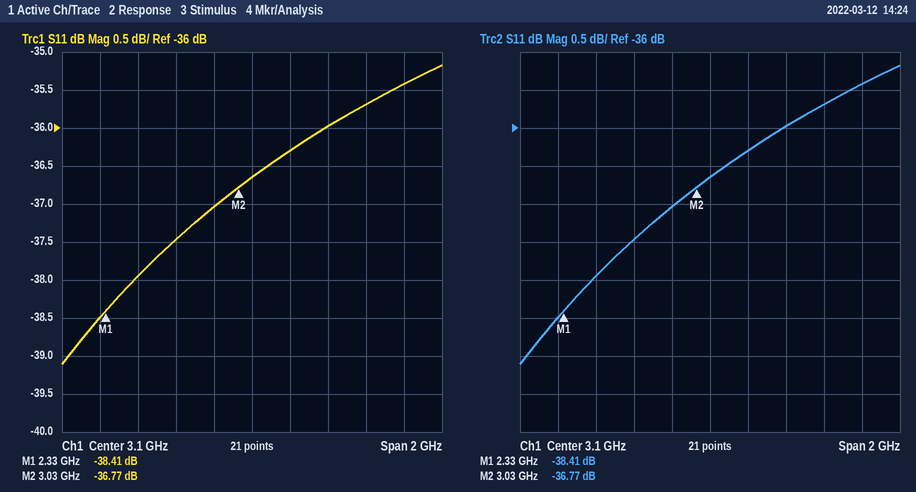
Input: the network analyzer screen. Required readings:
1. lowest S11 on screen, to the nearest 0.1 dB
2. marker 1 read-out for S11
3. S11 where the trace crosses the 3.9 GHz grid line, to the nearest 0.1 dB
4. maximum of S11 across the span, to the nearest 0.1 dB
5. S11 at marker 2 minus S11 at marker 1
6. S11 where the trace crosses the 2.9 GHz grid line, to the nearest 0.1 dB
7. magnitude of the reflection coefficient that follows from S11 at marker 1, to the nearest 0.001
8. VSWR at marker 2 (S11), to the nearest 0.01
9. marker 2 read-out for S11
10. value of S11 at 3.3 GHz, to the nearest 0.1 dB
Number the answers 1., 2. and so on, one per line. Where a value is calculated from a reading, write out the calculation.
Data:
1. -39.1 dB
2. -38.41 dB
3. -35.4 dB
4. -35.2 dB
5. -36.77 − (-38.41) = 1.64 dB
6. -37.0 dB
7. 10^(-38.41/20) ≈ 0.012
8. (1 + 0.0145)/(1 − 0.0145) ≈ 1.03
9. -36.77 dB
10. -36.3 dB
